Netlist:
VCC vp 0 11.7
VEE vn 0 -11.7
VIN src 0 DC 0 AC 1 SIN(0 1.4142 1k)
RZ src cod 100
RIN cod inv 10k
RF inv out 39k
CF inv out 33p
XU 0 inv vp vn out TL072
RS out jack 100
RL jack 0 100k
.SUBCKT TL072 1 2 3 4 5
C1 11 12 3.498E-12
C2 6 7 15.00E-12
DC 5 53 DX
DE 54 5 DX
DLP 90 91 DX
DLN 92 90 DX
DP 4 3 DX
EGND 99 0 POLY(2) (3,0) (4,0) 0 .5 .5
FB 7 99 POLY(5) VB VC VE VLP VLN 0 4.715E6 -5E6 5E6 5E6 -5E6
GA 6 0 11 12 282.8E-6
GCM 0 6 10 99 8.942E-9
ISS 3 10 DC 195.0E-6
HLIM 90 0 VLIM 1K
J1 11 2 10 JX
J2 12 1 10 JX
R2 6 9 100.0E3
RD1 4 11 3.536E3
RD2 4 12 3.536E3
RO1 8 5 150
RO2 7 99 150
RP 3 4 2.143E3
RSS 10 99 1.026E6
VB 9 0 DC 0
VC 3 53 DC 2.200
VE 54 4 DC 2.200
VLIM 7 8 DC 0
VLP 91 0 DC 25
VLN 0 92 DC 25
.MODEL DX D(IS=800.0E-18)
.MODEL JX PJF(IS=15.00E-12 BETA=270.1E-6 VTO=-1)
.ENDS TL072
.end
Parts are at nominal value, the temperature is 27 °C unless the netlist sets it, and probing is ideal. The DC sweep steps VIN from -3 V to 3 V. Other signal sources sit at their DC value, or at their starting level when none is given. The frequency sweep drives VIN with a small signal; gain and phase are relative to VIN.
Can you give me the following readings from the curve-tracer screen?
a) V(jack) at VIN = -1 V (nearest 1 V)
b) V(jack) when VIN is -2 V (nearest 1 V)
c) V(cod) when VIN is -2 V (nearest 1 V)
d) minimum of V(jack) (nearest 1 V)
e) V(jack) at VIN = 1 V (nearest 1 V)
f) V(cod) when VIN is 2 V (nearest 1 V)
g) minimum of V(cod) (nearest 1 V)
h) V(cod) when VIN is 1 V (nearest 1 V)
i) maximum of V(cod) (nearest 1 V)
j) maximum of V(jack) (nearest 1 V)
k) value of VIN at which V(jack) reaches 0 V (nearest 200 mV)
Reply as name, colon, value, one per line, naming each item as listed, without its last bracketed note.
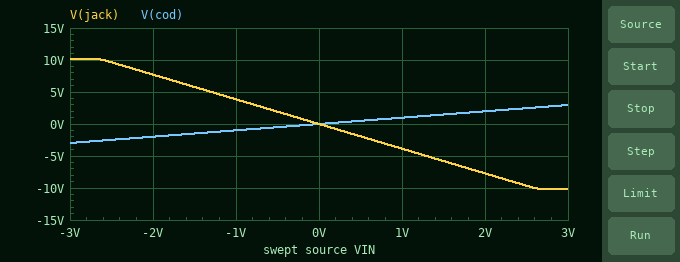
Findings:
V(jack) at VIN = -1 V: 4 V
V(jack) when VIN is -2 V: 8 V
V(cod) when VIN is -2 V: -2 V
minimum of V(jack): -10 V
V(jack) at VIN = 1 V: -4 V
V(cod) when VIN is 2 V: 2 V
minimum of V(cod): -3 V
V(cod) when VIN is 1 V: 1 V
maximum of V(cod): 3 V
maximum of V(jack): 10 V
value of VIN at which V(jack) reaches 0 V: 0 V
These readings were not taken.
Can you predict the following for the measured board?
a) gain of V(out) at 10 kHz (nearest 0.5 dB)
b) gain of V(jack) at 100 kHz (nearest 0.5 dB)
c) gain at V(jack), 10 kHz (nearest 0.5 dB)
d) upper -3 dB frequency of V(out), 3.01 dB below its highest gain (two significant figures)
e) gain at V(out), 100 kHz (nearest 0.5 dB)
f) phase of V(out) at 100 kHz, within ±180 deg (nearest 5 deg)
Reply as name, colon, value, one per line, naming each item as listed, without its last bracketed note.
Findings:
gain of V(out) at 10 kHz: 11.5 dB
gain of V(jack) at 100 kHz: 9.0 dB
gain at V(jack), 10 kHz: 11.5 dB
upper -3 dB frequency of V(out), 3.01 dB below its highest gain: 110 kHz
gain at V(out), 100 kHz: 9.0 dB
phase of V(out) at 100 kHz, within ±180 deg: 135 deg
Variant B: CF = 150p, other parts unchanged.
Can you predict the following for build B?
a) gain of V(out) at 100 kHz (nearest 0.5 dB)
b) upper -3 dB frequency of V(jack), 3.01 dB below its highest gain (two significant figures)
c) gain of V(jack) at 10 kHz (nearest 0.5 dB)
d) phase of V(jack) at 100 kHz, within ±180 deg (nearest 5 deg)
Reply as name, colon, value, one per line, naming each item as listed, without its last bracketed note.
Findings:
gain of V(out) at 100 kHz: 0 dB
upper -3 dB frequency of V(jack), 3.01 dB below its highest gain: 26 kHz
gain of V(jack) at 10 kHz: 11.0 dB
phase of V(jack) at 100 kHz, within ±180 deg: 105 deg
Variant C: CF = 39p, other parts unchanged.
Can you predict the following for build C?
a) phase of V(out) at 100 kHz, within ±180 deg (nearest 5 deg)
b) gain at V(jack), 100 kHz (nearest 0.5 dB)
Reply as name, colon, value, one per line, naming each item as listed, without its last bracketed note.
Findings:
phase of V(out) at 100 kHz, within ±180 deg: 130 deg
gain at V(jack), 100 kHz: 8.5 dB
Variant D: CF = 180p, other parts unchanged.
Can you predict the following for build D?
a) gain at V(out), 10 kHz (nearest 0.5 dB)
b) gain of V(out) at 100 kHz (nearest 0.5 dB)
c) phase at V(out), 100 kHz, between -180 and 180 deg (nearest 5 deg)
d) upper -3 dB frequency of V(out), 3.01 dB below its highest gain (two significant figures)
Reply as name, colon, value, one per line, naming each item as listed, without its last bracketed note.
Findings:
gain at V(out), 10 kHz: 11.0 dB
gain of V(out) at 100 kHz: -1.5 dB
phase at V(out), 100 kHz, between -180 and 180 deg: 100 deg
upper -3 dB frequency of V(out), 3.01 dB below its highest gain: 22 kHz
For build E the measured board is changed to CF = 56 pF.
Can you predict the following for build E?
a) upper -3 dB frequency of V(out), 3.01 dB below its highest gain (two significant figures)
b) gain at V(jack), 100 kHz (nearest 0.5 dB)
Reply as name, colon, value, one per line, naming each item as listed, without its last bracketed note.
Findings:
upper -3 dB frequency of V(out), 3.01 dB below its highest gain: 67 kHz
gain at V(jack), 100 kHz: 6.5 dB
